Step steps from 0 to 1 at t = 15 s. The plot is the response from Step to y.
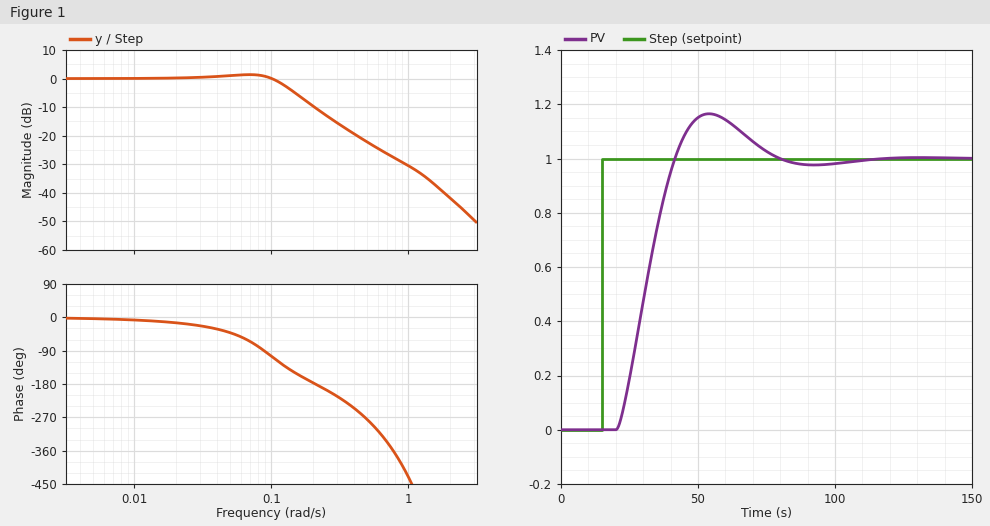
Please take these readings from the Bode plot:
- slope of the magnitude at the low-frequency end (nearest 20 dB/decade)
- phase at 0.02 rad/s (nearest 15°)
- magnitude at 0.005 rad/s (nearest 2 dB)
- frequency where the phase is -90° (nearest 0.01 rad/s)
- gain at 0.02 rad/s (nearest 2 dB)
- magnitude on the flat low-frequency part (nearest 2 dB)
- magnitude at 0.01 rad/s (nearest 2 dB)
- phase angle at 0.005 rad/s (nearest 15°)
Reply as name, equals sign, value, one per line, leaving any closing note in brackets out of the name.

slope of the magnitude at the low-frequency end = 0 dB/decade
phase at 0.02 rad/s = -15°
magnitude at 0.005 rad/s = 0 dB
frequency where the phase is -90° = 0.09 rad/s
gain at 0.02 rad/s = 0 dB
magnitude on the flat low-frequency part = 0 dB
magnitude at 0.01 rad/s = 0 dB
phase angle at 0.005 rad/s = 0°
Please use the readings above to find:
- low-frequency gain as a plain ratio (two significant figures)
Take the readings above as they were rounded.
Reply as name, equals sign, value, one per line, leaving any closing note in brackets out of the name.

low-frequency gain as a plain ratio = 1.0
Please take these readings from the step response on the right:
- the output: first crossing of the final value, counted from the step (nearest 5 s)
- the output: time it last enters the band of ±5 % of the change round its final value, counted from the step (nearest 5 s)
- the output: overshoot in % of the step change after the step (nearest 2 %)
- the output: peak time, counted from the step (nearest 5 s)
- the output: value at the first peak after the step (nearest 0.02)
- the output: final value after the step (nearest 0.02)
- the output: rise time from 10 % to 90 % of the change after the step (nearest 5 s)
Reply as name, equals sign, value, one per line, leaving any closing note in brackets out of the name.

the output: first crossing of the final value, counted from the step = 25 s
the output: time it last enters the band of ±5 % of the change round its final value, counted from the step = 55 s
the output: overshoot in % of the step change after the step = 16 %
the output: peak time, counted from the step = 40 s
the output: value at the first peak after the step = 1.16
the output: final value after the step = 1.00
the output: rise time from 10 % to 90 % of the change after the step = 15 s
